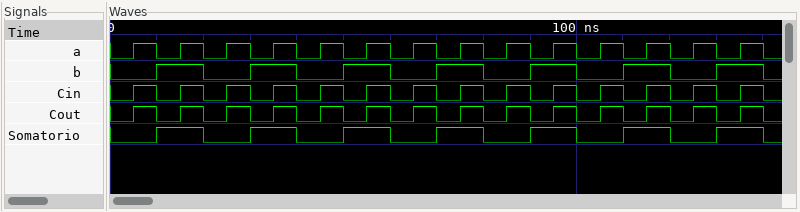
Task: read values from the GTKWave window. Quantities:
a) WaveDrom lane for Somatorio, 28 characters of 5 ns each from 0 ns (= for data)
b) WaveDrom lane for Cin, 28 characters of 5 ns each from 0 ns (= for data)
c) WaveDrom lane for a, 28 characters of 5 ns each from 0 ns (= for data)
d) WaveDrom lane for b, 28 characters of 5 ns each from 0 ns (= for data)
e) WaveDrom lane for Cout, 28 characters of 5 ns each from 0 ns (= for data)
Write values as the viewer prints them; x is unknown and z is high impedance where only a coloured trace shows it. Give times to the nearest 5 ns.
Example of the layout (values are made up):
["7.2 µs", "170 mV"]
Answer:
["{name: 'Somatorio', wave: '0.1.0.1.0.1.0.1.0.1.0.1.0.1.'}", "{name: 'Cin', wave: '0101010101010101010101010101'}", "{name: 'a', wave: '0101010101010101010101010101'}", "{name: 'b', wave: '0.1.0.1.0.1.0.1.0.1.0.1.0.1.'}", "{name: 'Cout', wave: '0101010101010101010101010101'}"]
